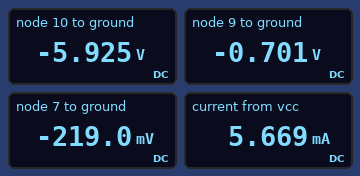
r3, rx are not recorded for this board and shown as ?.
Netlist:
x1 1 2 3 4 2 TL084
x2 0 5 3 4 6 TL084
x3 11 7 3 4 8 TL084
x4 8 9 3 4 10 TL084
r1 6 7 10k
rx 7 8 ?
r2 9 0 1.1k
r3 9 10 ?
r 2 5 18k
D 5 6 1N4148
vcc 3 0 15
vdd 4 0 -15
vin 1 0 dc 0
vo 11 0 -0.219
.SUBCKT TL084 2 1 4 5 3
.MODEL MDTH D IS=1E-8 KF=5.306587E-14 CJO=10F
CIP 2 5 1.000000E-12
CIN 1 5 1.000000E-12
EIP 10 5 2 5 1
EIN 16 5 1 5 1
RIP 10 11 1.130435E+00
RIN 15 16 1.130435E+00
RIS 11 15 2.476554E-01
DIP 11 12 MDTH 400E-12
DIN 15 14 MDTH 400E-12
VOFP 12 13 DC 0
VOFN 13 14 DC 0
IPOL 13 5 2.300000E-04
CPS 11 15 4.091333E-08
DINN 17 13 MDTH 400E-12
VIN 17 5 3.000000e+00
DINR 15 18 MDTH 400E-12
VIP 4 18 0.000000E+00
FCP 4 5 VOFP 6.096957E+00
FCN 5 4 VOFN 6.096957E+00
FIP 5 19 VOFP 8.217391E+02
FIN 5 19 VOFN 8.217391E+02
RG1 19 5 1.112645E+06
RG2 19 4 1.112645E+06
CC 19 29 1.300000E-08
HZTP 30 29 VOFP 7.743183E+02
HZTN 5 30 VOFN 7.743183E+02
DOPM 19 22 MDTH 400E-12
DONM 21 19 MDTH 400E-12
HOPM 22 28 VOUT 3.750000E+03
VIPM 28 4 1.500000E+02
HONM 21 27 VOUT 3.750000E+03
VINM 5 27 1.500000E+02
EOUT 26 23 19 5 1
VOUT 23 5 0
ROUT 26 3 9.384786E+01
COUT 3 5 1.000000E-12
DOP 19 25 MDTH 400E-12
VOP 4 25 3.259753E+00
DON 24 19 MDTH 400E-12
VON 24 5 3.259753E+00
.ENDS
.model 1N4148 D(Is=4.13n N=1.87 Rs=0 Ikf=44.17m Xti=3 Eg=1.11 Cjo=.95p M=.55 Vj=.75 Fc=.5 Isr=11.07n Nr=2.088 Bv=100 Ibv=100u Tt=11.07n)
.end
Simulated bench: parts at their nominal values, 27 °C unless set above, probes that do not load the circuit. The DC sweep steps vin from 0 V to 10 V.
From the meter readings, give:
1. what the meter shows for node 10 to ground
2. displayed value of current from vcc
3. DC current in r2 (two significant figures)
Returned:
-5.925 V
5.669 mA
640 µA
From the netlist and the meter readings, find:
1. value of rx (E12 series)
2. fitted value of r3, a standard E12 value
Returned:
22 kΩ
8.2 kΩ
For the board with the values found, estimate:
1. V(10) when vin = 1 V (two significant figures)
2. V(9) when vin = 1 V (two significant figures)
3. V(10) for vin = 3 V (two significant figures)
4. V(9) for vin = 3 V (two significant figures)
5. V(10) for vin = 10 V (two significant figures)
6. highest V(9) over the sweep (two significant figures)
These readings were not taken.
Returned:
2.2 V
260 mV
3.3 V
390 mV
4.5 V
530 mV
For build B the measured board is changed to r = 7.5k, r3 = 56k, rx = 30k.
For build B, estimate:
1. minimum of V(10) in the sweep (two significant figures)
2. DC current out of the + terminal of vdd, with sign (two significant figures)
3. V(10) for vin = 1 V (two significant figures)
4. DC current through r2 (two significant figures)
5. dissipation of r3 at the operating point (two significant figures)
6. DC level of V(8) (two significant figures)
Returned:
-13 V
-5.9 mA
13 V
220 µA
2.8 mW
-880 mV
